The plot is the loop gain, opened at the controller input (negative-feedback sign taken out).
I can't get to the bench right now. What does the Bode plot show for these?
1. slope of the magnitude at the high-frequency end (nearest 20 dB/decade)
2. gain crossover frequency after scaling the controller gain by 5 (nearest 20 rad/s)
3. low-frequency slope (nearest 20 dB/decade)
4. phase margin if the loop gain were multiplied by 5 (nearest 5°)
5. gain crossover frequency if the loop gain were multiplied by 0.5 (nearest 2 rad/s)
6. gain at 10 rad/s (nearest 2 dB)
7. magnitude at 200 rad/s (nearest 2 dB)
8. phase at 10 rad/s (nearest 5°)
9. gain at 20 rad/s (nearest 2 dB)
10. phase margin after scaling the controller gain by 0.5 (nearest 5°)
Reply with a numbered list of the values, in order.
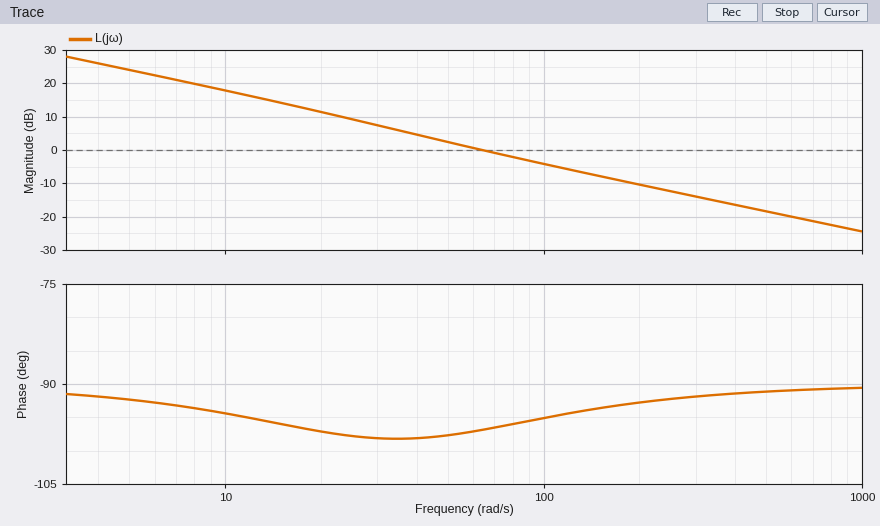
1. -20 dB/decade
2. 300 rad/s
3. -20 dB/decade
4. 90°
5. 34 rad/s
6. 18 dB
7. -10 dB
8. -95°
9. 12 dB
10. 80°
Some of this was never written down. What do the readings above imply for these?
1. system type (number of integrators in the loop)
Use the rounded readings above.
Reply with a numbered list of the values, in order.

1. 1
